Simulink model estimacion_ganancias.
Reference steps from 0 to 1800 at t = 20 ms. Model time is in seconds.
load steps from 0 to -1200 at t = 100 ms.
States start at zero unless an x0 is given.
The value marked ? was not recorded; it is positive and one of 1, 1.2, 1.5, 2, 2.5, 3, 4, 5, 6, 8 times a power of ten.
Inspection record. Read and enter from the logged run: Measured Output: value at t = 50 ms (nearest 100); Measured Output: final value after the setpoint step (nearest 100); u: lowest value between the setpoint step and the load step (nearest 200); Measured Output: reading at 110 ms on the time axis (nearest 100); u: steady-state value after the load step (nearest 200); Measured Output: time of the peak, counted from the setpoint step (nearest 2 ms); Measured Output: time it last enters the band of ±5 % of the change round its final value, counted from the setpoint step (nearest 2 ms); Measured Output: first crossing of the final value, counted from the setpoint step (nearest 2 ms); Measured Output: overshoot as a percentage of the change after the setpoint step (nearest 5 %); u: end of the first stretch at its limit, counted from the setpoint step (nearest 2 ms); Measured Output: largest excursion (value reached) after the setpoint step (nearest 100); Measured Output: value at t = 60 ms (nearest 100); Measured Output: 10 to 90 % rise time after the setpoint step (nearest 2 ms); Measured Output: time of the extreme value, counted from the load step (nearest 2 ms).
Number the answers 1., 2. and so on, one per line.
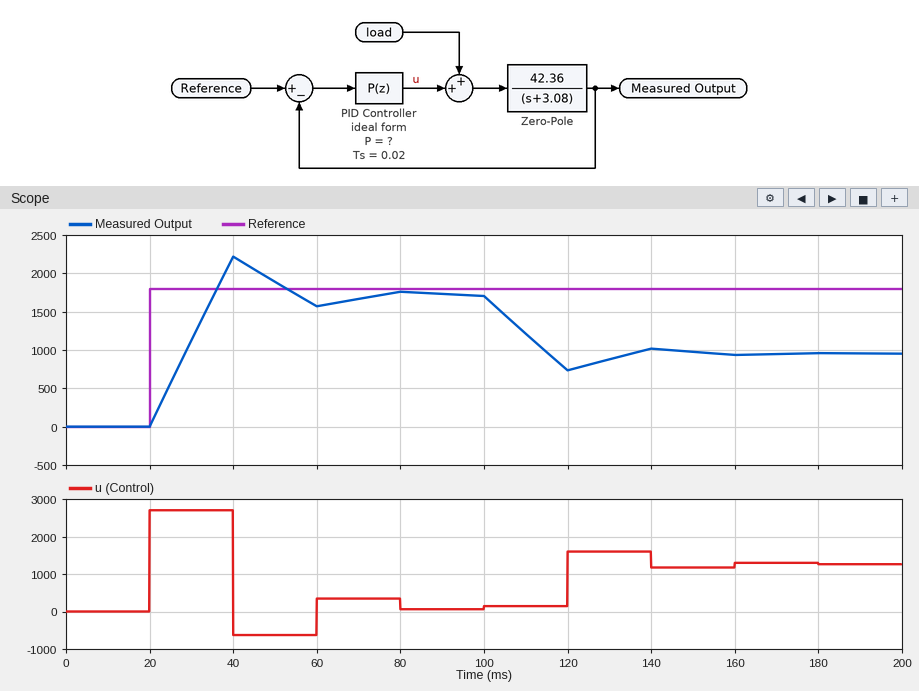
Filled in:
1. 1900
2. 1700
3. -600
4. 1200
5. 1200
6. 20 ms
7. 46 ms
8. 16 ms
9. 30 %
10. 20 ms
11. 2200
12. 1600
13. 12 ms
14. 20 ms
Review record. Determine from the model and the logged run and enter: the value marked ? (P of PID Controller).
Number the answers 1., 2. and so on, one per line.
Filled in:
1. 1.5
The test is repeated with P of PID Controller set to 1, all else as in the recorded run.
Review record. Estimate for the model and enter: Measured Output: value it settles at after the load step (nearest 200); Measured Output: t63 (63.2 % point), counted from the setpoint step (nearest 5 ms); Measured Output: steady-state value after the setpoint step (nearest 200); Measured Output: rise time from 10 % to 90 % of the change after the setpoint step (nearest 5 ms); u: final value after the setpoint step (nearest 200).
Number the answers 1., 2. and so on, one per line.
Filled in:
1. 600
2. 15 ms
3. 1600
4. 20 ms
5. 200
